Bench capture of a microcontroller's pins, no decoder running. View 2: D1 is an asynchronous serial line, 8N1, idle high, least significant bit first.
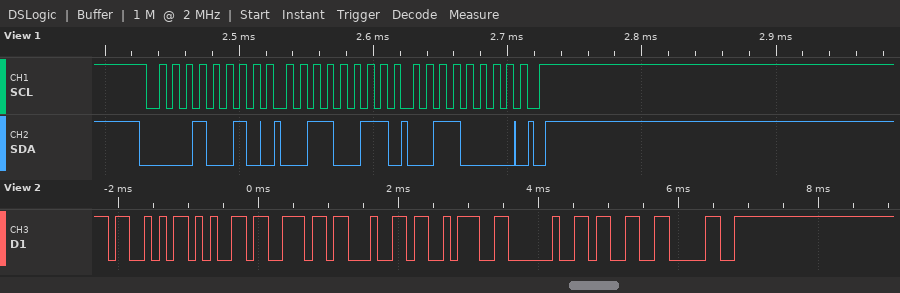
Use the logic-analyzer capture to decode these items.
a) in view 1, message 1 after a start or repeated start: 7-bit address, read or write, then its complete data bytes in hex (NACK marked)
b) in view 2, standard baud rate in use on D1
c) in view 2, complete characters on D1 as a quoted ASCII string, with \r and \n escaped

0x09 write: 33 30
9600 baud
"Send: 30"
